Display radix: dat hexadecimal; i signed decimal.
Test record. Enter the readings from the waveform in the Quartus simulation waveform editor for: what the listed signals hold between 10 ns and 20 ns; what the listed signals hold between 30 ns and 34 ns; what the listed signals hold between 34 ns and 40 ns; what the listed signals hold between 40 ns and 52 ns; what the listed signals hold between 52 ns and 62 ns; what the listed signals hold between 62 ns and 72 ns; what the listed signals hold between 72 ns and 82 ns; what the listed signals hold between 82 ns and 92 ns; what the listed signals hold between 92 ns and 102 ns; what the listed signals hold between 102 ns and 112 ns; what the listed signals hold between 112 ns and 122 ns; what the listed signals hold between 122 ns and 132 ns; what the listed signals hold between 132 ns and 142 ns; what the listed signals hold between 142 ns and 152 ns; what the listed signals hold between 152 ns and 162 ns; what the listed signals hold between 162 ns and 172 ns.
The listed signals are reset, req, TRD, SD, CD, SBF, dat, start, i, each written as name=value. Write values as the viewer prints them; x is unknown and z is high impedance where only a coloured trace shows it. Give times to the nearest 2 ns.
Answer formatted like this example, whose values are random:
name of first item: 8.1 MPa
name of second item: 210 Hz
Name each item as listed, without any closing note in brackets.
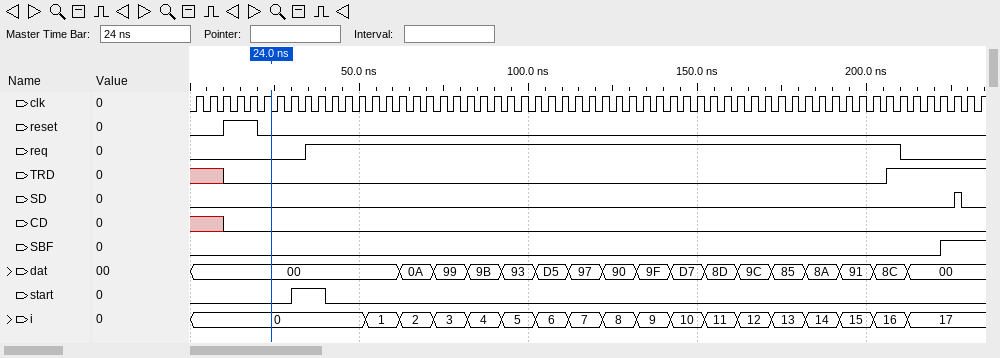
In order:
what the listed signals hold between 10 ns and 20 ns: reset=1, req=0, TRD=0, SD=0, CD=0, SBF=0, dat=00, start=0, i=0
what the listed signals hold between 30 ns and 34 ns: reset=0, req=0, TRD=0, SD=0, CD=0, SBF=0, dat=00, start=1, i=0
what the listed signals hold between 34 ns and 40 ns: reset=0, req=1, TRD=0, SD=0, CD=0, SBF=0, dat=00, start=1, i=0
what the listed signals hold between 40 ns and 52 ns: reset=0, req=1, TRD=0, SD=0, CD=0, SBF=0, dat=00, start=0, i=0
what the listed signals hold between 52 ns and 62 ns: reset=0, req=1, TRD=0, SD=0, CD=0, SBF=0, dat=00, start=0, i=1
what the listed signals hold between 62 ns and 72 ns: reset=0, req=1, TRD=0, SD=0, CD=0, SBF=0, dat=0A, start=0, i=2
what the listed signals hold between 72 ns and 82 ns: reset=0, req=1, TRD=0, SD=0, CD=0, SBF=0, dat=99, start=0, i=3
what the listed signals hold between 82 ns and 92 ns: reset=0, req=1, TRD=0, SD=0, CD=0, SBF=0, dat=9B, start=0, i=4
what the listed signals hold between 92 ns and 102 ns: reset=0, req=1, TRD=0, SD=0, CD=0, SBF=0, dat=93, start=0, i=5
what the listed signals hold between 102 ns and 112 ns: reset=0, req=1, TRD=0, SD=0, CD=0, SBF=0, dat=D5, start=0, i=6
what the listed signals hold between 112 ns and 122 ns: reset=0, req=1, TRD=0, SD=0, CD=0, SBF=0, dat=97, start=0, i=7
what the listed signals hold between 122 ns and 132 ns: reset=0, req=1, TRD=0, SD=0, CD=0, SBF=0, dat=90, start=0, i=8
what the listed signals hold between 132 ns and 142 ns: reset=0, req=1, TRD=0, SD=0, CD=0, SBF=0, dat=9F, start=0, i=9
what the listed signals hold between 142 ns and 152 ns: reset=0, req=1, TRD=0, SD=0, CD=0, SBF=0, dat=D7, start=0, i=10
what the listed signals hold between 152 ns and 162 ns: reset=0, req=1, TRD=0, SD=0, CD=0, SBF=0, dat=8D, start=0, i=11
what the listed signals hold between 162 ns and 172 ns: reset=0, req=1, TRD=0, SD=0, CD=0, SBF=0, dat=9C, start=0, i=12
